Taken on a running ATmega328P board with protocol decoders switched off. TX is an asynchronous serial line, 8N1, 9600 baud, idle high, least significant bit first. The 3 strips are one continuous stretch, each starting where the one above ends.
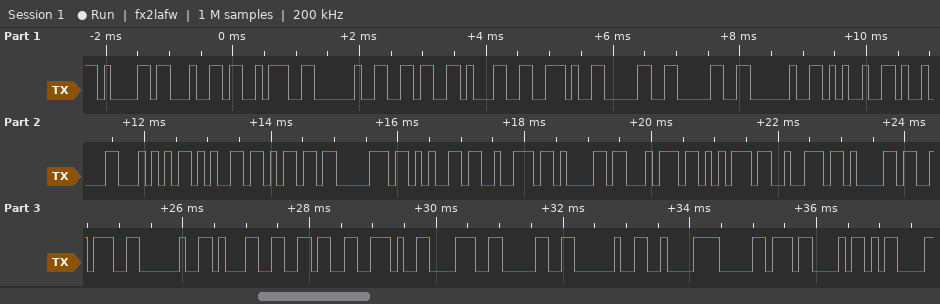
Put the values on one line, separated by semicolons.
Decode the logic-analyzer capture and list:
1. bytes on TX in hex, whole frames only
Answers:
61 64 3A 20 36 31 2E 30 30 20 25 09 54 65 6D 70 65 72 61 74 75 72 61 3A 20 31 36 2E 38 30 20 C2 B0 43 0D
